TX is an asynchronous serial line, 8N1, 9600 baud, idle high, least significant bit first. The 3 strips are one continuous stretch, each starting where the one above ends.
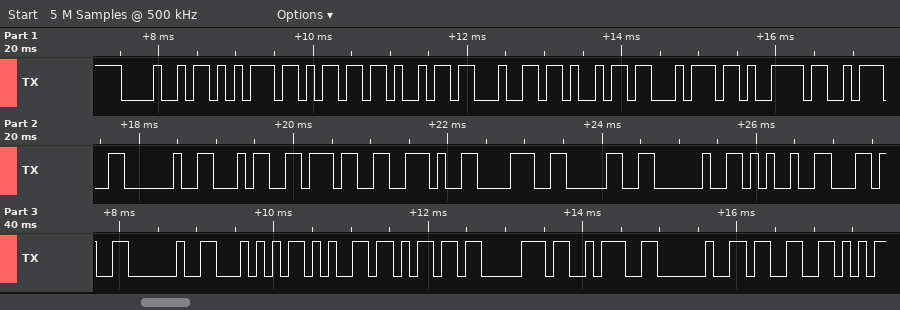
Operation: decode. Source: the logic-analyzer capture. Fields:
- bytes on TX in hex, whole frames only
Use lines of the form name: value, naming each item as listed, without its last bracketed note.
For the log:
bytes on TX in hex, whole frames only: 48 75 6D 69 64 69 74 79 3A 20 34 37 2E 38 30 20 25 2C 20 54 65 6D 70 3A 20 33
